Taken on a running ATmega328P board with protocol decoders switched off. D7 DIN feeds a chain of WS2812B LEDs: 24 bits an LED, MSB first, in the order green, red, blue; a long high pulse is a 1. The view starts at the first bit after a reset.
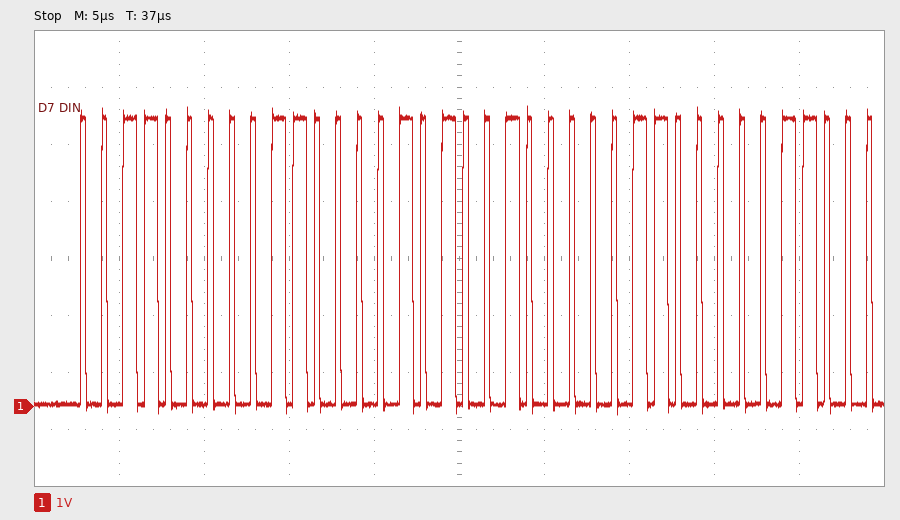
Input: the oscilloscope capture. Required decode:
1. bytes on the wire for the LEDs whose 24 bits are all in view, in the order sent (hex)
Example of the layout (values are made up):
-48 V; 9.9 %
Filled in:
30 61 48
